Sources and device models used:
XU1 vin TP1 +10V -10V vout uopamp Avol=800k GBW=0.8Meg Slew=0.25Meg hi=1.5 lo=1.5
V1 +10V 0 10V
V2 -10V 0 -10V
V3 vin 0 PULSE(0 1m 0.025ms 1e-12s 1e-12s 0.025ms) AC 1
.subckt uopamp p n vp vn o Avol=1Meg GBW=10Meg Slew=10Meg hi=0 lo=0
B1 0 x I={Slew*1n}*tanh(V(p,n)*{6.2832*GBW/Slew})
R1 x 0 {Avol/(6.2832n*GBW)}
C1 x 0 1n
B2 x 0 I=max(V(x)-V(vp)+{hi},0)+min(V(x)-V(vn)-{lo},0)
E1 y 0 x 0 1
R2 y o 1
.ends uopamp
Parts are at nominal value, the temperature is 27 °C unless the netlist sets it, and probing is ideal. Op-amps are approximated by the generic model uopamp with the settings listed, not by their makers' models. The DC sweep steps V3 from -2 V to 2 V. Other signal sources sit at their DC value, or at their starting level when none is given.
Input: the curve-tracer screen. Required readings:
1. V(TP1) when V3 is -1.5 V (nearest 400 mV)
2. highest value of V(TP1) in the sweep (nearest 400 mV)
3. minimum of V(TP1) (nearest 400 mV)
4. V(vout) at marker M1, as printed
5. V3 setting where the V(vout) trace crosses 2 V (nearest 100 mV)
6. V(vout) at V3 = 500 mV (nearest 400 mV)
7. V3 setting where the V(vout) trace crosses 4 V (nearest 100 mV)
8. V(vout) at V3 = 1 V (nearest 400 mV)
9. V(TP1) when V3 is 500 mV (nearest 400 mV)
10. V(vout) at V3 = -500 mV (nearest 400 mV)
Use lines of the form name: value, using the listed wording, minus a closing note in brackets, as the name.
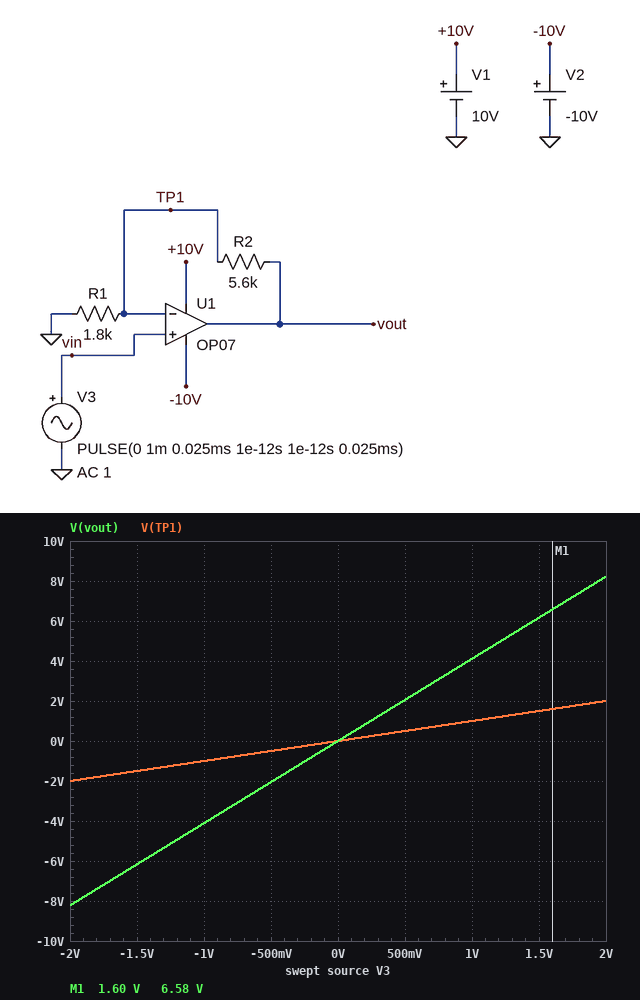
V(TP1) when V3 is -1.5 V: -1.6 V
highest value of V(TP1) in the sweep: 2.0 V
minimum of V(TP1): -2.0 V
V(vout) at marker M1, as printed: 6.58 V
V3 setting where the V(vout) trace crosses 2 V: 500 mV
V(vout) at V3 = 500 mV: 2.0 V
V3 setting where the V(vout) trace crosses 4 V: 1.0 V
V(vout) at V3 = 1 V: 4.0 V
V(TP1) when V3 is 500 mV: 400 mV
V(vout) at V3 = -500 mV: -2.0 V
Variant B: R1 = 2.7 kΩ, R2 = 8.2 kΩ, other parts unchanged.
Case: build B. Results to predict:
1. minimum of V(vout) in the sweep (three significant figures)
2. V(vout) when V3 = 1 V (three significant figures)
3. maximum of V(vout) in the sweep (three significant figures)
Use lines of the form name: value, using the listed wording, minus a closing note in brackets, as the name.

minimum of V(vout) in the sweep: -8.07 V
V(vout) when V3 = 1 V: 4.04 V
maximum of V(vout) in the sweep: 8.07 V
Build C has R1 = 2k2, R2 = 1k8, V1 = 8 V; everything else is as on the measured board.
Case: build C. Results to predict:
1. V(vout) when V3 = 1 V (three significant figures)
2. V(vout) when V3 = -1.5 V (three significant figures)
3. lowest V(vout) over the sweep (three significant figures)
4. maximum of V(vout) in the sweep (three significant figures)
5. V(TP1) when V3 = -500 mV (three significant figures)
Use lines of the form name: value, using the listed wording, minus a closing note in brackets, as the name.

V(vout) when V3 = 1 V: 1.82 V
V(vout) when V3 = -1.5 V: -2.73 V
lowest V(vout) over the sweep: -3.64 V
maximum of V(vout) in the sweep: 3.64 V
V(TP1) when V3 = -500 mV: -500 mV
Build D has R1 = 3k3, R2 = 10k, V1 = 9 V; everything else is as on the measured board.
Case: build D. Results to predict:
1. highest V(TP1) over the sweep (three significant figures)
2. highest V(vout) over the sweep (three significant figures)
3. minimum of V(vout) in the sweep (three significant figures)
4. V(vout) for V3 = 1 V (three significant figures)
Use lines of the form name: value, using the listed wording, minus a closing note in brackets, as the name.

highest V(TP1) over the sweep: 1.86 V
highest V(vout) over the sweep: 7.50 V
minimum of V(vout) in the sweep: -8.06 V
V(vout) for V3 = 1 V: 4.03 V
